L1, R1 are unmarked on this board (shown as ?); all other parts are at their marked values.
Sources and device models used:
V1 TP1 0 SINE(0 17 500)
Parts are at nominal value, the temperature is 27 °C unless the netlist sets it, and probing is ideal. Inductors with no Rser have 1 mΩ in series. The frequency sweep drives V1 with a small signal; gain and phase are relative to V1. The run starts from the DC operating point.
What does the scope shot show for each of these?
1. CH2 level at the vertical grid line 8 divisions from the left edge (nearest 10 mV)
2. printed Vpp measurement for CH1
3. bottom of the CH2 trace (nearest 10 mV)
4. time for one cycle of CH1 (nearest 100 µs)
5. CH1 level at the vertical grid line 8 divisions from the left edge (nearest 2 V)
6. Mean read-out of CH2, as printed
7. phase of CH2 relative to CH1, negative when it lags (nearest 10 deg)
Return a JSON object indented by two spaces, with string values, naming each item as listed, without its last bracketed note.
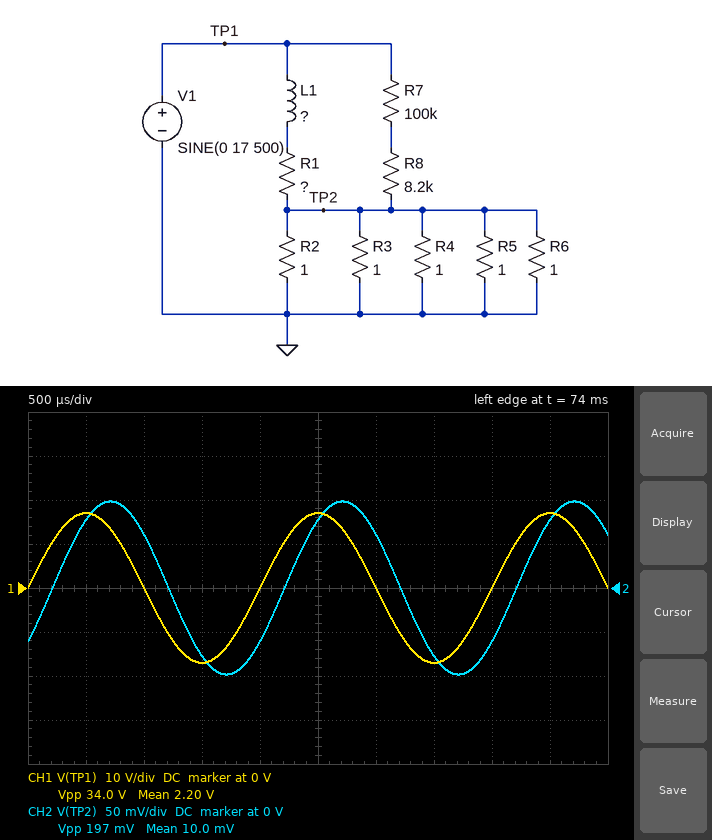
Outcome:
{
  "CH2 level at the vertical grid line 8 divisions from the left edge": "-60 mV",
  "printed Vpp measurement for CH1": "34.0 V",
  "bottom of the CH2 trace": "-100 mV",
  "time for one cycle of CH1": "2.0 ms",
  "CH1 level at the vertical grid line 8 divisions from the left edge": "0 V",
  "Mean read-out of CH2, as printed": "10.0 mV",
  "phase of CH2 relative to CH1, negative when it lags": "-40 deg"
}
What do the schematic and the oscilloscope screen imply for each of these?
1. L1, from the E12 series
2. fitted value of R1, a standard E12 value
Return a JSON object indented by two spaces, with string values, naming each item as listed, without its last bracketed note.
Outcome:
{
  "L1, from the E12 series": "6.8 mH",
  "fitted value of R1, a standard E12 value": "27 Ω"
}
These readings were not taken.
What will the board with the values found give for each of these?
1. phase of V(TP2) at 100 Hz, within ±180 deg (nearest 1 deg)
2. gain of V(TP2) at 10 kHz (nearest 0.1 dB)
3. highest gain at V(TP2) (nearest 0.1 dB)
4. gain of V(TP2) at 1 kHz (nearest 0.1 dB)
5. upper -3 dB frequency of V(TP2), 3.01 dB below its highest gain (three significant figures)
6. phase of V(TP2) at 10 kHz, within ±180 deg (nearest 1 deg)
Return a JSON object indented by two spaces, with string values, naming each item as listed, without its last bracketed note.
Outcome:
{
  "phase of V(TP2) at 100 Hz, within ±180 deg": "-9 deg",
  "gain of V(TP2) at 10 kHz": "-66.6 dB",
  "highest gain at V(TP2)": "-42.7 dB",
  "gain of V(TP2) at 1 kHz": "-48.1 dB",
  "upper -3 dB frequency of V(TP2), 3.01 dB below its highest gain": "637 Hz",
  "phase of V(TP2) at 10 kHz, within ±180 deg": "-86 deg"
}
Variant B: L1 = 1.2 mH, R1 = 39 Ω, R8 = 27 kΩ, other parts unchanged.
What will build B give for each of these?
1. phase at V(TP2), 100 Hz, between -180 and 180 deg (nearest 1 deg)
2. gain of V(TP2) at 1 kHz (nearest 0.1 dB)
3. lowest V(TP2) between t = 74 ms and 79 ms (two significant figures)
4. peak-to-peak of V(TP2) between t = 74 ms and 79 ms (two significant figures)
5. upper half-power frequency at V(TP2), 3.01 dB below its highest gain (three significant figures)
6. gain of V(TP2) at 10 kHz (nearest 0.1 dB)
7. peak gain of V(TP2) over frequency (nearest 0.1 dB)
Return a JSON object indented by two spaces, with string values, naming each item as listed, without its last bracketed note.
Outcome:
{
  "phase at V(TP2), 100 Hz, between -180 and 180 deg": "-1 deg",
  "gain of V(TP2) at 1 kHz": "-46.0 dB",
  "lowest V(TP2) between t = 74 ms and 79 ms": "-86 mV",
  "peak-to-peak of V(TP2) between t = 74 ms and 79 ms": "170 mV",
  "upper half-power frequency at V(TP2), 3.01 dB below its highest gain": "5.20 kHz",
  "gain of V(TP2) at 10 kHz": "-52.6 dB",
  "peak gain of V(TP2) over frequency": "-45.8 dB"
}
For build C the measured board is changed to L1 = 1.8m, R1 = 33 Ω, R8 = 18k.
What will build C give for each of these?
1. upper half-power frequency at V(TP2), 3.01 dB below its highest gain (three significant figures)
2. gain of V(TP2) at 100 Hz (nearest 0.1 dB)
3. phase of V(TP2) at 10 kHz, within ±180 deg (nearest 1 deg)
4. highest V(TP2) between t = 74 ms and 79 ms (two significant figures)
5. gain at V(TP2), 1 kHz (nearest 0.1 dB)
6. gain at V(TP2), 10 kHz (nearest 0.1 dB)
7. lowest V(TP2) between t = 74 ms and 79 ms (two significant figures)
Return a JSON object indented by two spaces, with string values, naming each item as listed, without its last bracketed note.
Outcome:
{
  "upper half-power frequency at V(TP2), 3.01 dB below its highest gain": "2.94 kHz",
  "gain of V(TP2) at 100 Hz": "-44.4 dB",
  "phase of V(TP2) at 10 kHz, within ±180 deg": "-74 deg",
  "highest V(TP2) between t = 74 ms and 79 ms": "100 mV",
  "gain at V(TP2), 1 kHz": "-44.9 dB",
  "gain at V(TP2), 10 kHz": "-55.4 dB",
  "lowest V(TP2) between t = 74 ms and 79 ms": "-100 mV"
}
